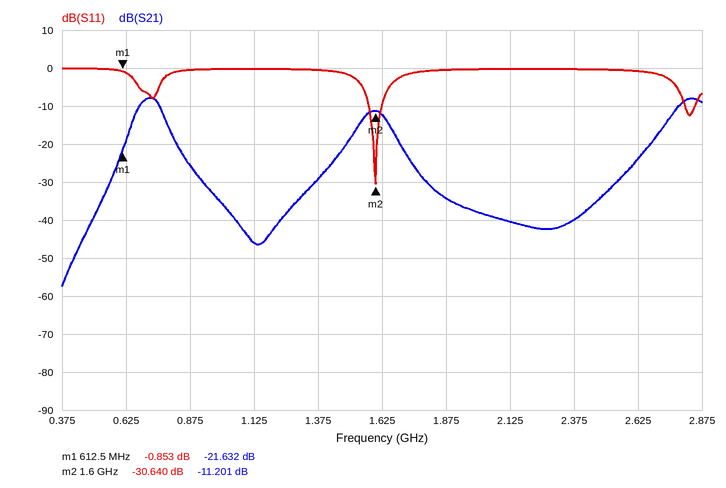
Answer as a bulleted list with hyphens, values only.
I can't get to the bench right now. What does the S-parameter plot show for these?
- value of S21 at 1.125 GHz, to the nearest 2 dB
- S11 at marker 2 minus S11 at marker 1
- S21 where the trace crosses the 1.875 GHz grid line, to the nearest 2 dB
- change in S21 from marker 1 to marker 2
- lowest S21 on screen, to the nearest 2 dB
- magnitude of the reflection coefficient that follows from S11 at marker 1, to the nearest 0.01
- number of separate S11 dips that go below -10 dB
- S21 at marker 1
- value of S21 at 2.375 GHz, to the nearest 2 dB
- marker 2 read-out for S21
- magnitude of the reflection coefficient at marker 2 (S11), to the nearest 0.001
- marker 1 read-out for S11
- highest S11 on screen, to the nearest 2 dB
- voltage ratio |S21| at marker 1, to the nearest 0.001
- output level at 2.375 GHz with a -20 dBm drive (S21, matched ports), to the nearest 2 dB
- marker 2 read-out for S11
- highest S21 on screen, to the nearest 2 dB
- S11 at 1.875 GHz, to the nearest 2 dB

- -46 dB
- -29.787 dB
- -34 dB
- 10.431 dB
- -58 dB
- 0.91
- 2
- -21.632 dB
- -40 dB
- -11.201 dB
- 0.029
- -0.853 dB
- 0 dB
- 0.083
- -60 dBm
- -30.640 dB
- -8 dB
- 0 dB
